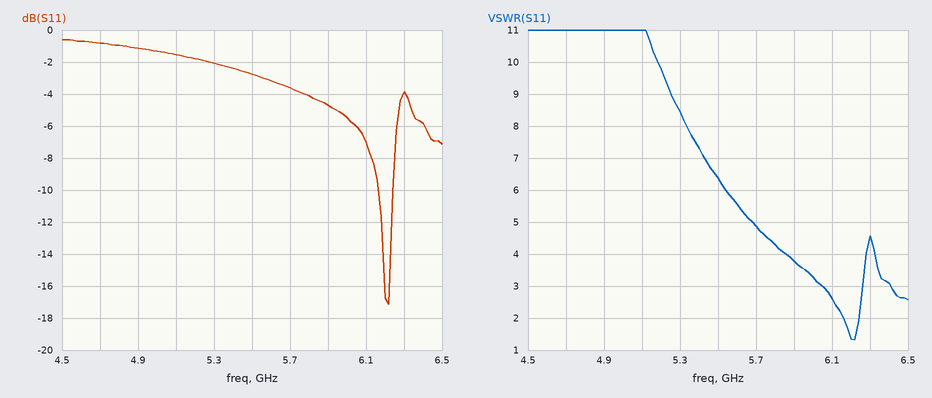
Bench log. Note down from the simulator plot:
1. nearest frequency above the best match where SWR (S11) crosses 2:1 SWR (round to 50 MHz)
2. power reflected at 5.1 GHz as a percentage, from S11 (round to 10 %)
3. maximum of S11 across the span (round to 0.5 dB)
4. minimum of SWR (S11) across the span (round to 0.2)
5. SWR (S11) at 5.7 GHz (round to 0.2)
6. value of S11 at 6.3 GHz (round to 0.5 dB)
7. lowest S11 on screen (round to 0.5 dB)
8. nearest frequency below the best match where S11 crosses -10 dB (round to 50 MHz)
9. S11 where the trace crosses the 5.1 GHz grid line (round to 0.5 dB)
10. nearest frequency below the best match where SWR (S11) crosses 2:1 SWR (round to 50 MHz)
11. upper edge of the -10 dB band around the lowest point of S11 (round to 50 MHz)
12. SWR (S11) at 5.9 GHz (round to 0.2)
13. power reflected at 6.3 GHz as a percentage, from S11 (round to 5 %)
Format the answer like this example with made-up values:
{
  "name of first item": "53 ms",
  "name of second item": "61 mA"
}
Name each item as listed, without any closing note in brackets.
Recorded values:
{
  "nearest frequency above the best match where SWR (S11) crosses 2:1 SWR": "6.25 GHz",
  "power reflected at 5.1 GHz as a percentage, from S11": "70 %",
  "maximum of S11 across the span": "-0.5 dB",
  "minimum of SWR (S11) across the span": "1.4",
  "SWR (S11) at 5.7 GHz": "4.8",
  "value of S11 at 6.3 GHz": "-4.0 dB",
  "lowest S11 on screen": "-17.0 dB",
  "nearest frequency below the best match where S11 crosses -10 dB": "6.15 GHz",
  "S11 where the trace crosses the 5.1 GHz grid line": "-1.5 dB",
  "nearest frequency below the best match where SWR (S11) crosses 2:1 SWR": "6.15 GHz",
  "upper edge of the -10 dB band around the lowest point of S11": "6.25 GHz",
  "SWR (S11) at 5.9 GHz": "3.8",
  "power reflected at 6.3 GHz as a percentage, from S11": "40 %"
}
